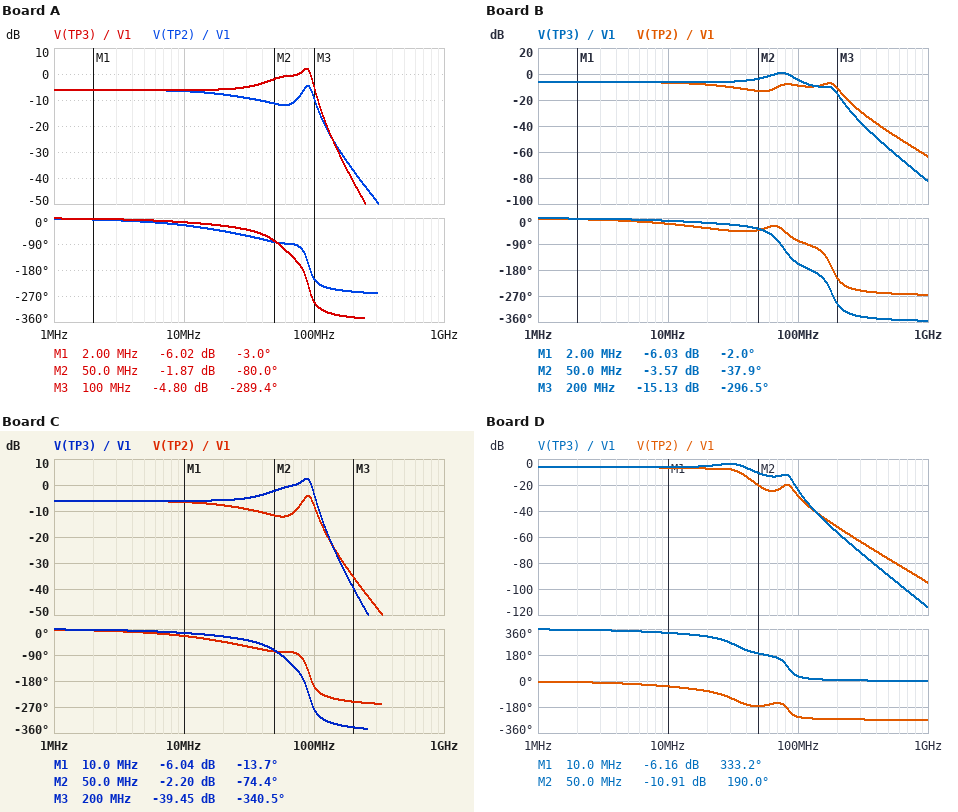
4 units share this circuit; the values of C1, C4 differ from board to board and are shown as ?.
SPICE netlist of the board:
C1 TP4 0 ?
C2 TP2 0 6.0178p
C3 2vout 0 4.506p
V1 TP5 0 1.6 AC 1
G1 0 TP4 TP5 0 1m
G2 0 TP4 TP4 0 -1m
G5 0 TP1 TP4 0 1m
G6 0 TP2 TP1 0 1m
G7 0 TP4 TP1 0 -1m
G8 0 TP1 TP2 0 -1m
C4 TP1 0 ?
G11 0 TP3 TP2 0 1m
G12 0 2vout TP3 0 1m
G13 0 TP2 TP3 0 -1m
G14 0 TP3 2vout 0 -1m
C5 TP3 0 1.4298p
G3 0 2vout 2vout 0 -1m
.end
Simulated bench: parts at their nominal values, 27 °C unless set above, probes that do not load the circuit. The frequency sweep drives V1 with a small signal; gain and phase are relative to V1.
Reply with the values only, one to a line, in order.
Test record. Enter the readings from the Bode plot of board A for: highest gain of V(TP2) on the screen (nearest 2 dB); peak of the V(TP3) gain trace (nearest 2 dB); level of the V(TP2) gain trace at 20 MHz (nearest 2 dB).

-4 dB
2 dB
-8 dB
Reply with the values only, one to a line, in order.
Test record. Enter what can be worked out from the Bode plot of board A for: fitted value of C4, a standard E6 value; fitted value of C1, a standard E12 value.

2.2 pF
3.3 pF
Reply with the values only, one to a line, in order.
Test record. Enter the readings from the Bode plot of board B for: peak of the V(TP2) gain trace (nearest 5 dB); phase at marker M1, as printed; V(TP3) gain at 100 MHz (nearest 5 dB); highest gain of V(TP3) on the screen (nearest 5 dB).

-5 dB
-2.0 deg
-5 dB
0 dB
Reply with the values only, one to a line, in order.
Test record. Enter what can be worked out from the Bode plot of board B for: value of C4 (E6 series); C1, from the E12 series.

470 fF
2.2 pF
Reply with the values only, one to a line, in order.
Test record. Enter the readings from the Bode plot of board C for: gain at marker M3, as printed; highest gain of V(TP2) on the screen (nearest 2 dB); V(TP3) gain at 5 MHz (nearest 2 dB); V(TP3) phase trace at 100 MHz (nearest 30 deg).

-39.45 dB
-4 dB
-6 dB
-270 deg
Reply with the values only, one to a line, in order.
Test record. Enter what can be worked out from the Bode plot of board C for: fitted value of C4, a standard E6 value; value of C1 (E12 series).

2.2 pF
2.7 pF
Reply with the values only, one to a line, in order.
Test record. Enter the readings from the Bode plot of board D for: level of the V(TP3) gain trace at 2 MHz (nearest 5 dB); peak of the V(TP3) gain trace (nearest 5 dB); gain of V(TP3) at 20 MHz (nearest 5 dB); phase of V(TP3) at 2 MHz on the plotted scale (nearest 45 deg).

-5 dB
-5 dB
-5 dB
360 deg
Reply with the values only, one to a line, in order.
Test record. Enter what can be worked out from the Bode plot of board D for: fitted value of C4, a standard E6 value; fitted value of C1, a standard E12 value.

4.7 pF
8.2 pF
